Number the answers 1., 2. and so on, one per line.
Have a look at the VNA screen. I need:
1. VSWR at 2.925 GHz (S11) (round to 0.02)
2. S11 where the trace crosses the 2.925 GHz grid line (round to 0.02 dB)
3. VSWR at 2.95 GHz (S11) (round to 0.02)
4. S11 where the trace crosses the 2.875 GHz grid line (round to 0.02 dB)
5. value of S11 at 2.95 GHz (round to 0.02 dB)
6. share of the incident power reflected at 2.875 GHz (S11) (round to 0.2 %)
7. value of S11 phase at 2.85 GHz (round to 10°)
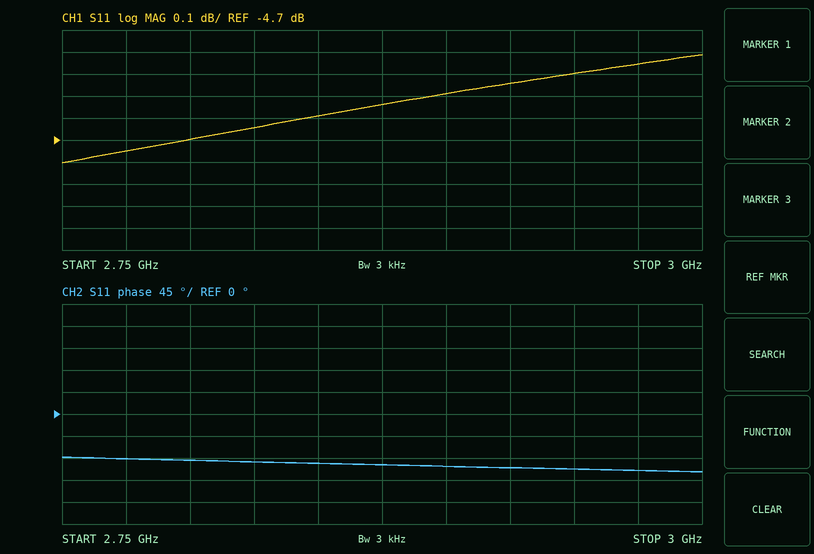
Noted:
1. 4.00
2. -4.44 dB
3. 4.04
4. -4.54 dB
5. -4.40 dB
6. 35.2 %
7. -100°
